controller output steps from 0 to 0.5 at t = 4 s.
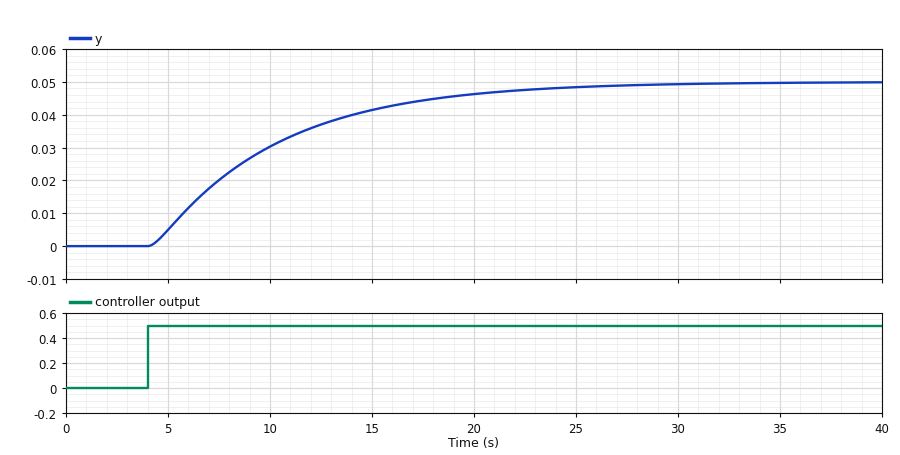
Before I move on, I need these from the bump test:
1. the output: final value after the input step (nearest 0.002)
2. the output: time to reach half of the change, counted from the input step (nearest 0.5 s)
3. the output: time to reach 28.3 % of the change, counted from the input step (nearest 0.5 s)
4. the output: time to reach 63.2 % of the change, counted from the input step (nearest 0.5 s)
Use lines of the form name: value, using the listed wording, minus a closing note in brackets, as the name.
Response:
the output: final value after the input step: 0.050
the output: time to reach half of the change, counted from the input step: 4.5 s
the output: time to reach 28.3 % of the change, counted from the input step: 2.5 s
the output: time to reach 63.2 % of the change, counted from the input step: 6.5 s
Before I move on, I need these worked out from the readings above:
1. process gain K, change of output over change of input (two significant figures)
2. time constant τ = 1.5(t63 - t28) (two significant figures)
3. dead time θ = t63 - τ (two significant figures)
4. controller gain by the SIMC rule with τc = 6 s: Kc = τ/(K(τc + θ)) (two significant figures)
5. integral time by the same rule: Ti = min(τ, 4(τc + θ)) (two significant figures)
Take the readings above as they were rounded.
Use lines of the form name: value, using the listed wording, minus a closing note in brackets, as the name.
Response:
process gain K, change of output over change of input: 0.10
time constant τ = 1.5(t63 - t28): 6.0 s
dead time θ = t63 - τ: 0.50 s
controller gain by the SIMC rule with τc = 6 s: Kc = τ/(K(τc + θ)): 9.2
integral time by the same rule: Ti = min(τ, 4(τc + θ)): 6.0 s
